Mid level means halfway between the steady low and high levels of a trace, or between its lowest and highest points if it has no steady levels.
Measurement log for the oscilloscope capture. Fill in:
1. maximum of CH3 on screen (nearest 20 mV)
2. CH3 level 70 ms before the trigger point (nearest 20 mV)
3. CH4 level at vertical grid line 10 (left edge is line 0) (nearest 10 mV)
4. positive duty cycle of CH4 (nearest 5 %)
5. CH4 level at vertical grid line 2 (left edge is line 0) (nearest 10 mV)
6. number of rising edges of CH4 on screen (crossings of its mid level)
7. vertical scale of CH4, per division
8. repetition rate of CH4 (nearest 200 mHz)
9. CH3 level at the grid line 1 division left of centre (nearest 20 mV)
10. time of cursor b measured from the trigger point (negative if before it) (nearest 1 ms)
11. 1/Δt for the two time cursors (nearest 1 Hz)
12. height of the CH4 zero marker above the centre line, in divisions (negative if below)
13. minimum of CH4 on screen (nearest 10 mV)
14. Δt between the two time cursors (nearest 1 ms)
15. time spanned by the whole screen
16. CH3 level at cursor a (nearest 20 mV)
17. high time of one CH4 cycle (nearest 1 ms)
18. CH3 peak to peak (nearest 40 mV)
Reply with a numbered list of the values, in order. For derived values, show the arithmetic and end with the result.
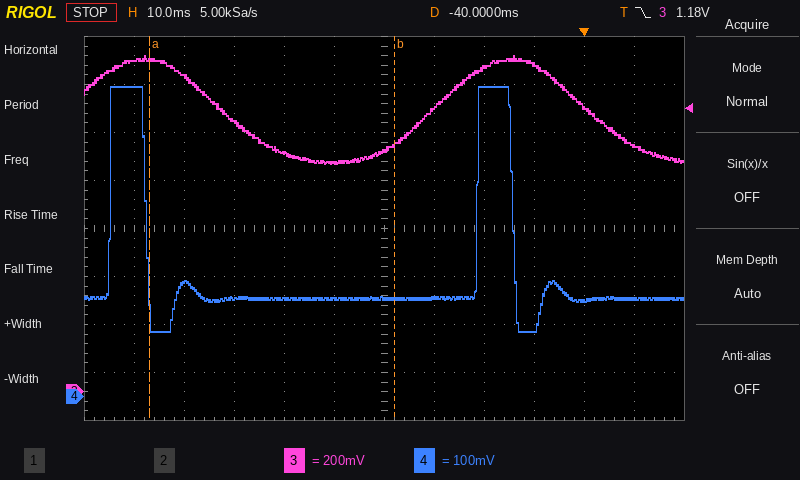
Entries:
1. 1.40 V
2. 1.12 V
3. 200 mV
4. 10 %
5. 240 mV
6. 2
7. 100 mV
8. 13.6 Hz
9. 960 mV
10. -38 ms
11. 1 / 49 ms ≈ 20 Hz
12. -3.5 div
13. 140 mV
14. 49 ms
15. 120 ms
16. 1.38 V
17. 7 ms
18. 440 mV
